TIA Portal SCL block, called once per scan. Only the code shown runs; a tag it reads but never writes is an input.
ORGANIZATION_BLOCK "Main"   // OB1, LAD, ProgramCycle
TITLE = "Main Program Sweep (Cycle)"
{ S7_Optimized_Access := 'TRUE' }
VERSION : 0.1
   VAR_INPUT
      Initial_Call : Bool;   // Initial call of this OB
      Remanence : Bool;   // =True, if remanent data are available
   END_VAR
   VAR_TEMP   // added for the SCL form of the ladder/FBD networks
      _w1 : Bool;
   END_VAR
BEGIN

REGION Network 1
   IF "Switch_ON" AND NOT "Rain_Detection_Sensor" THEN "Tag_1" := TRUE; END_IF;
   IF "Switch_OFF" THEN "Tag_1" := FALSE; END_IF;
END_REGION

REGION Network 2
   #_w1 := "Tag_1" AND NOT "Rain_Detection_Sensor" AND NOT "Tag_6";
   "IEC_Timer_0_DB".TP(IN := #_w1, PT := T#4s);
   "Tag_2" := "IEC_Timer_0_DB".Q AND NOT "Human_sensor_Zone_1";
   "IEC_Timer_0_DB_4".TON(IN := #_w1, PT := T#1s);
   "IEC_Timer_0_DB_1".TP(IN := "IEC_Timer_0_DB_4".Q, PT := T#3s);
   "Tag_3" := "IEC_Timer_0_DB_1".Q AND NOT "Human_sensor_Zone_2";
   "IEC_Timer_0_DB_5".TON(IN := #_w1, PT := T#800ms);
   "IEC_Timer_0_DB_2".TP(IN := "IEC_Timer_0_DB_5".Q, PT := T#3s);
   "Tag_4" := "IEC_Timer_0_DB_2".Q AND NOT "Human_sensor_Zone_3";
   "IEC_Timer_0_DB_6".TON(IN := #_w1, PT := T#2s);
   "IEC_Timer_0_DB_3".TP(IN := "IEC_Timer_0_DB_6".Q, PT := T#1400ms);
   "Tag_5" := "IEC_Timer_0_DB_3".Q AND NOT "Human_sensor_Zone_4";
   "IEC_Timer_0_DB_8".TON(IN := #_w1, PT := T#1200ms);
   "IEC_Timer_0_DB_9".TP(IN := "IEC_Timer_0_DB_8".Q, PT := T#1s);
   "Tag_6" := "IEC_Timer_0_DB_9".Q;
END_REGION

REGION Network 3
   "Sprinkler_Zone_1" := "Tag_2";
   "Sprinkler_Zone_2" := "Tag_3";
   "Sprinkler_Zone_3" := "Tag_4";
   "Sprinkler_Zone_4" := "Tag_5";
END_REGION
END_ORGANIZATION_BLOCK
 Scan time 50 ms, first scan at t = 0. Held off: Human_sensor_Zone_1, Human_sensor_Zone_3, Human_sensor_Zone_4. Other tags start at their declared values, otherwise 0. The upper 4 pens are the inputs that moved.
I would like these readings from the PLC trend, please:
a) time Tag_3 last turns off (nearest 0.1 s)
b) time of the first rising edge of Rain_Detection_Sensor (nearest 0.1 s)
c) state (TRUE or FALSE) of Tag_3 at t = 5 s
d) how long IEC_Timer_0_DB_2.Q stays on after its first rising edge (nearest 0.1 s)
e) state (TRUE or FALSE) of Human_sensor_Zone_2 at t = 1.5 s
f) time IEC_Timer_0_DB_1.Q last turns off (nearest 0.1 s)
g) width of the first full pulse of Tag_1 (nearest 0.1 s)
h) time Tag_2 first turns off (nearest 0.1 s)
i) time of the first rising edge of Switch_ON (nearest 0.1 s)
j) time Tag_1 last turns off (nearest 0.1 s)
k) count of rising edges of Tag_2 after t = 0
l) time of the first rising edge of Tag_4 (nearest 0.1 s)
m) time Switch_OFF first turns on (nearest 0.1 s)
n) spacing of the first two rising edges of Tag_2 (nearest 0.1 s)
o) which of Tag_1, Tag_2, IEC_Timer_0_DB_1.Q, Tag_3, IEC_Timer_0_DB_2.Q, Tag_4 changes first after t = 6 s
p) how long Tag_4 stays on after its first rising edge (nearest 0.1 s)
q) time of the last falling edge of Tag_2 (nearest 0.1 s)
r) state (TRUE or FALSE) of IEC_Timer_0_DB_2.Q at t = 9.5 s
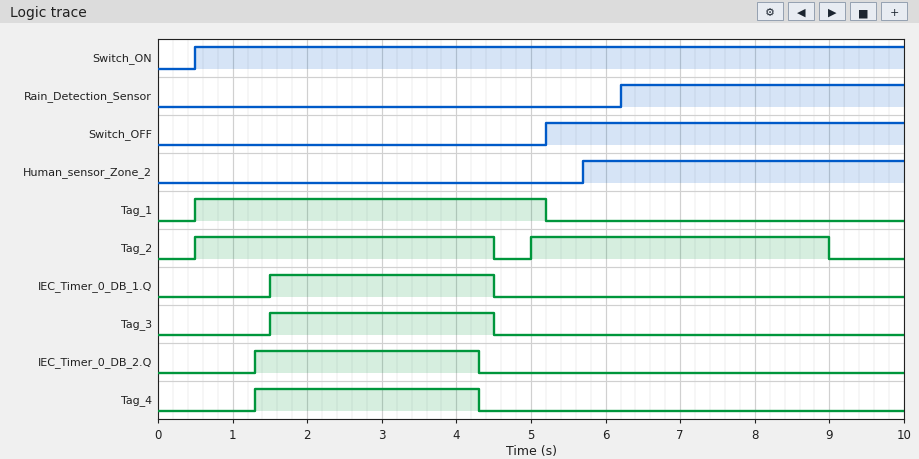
4.5 s
6.2 s
FALSE
3.0 s
FALSE
4.5 s
4.7 s
4.5 s
0.5 s
5.2 s
2
1.3 s
5.2 s
4.5 s
Tag_2
3.0 s
9.0 s
FALSE
